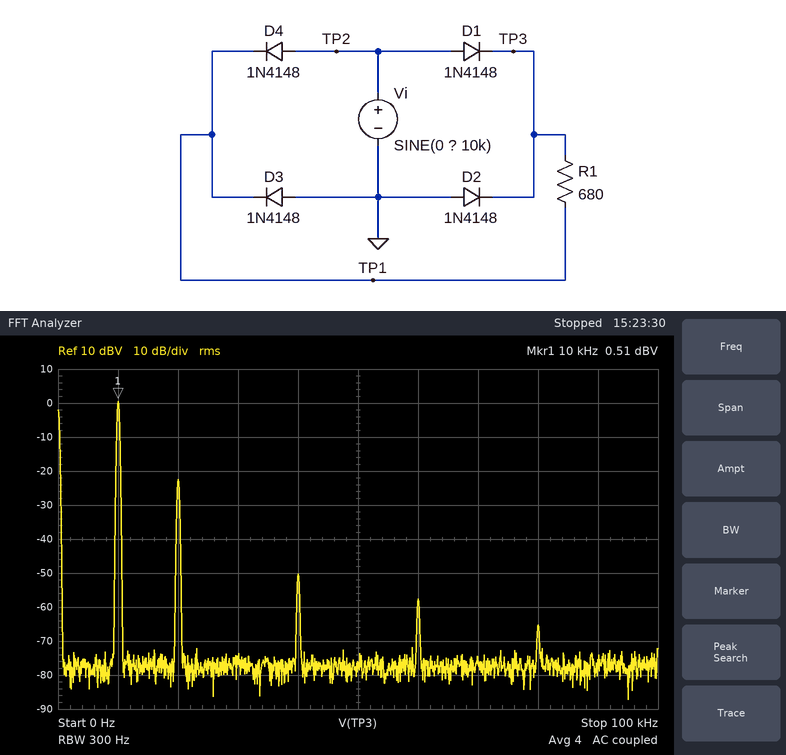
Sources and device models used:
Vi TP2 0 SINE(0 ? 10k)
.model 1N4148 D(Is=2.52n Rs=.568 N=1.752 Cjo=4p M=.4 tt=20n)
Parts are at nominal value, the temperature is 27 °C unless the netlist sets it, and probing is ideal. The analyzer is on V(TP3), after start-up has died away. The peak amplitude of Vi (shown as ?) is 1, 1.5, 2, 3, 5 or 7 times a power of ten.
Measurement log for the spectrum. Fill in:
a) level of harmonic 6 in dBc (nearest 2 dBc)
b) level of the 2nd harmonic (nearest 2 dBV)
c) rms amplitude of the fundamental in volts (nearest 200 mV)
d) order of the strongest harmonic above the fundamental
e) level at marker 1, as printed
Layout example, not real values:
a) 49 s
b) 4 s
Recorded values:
a) -58 dBc
b) -22 dBV
c) 1.0 V
d) 2
e) 0.51 dBV
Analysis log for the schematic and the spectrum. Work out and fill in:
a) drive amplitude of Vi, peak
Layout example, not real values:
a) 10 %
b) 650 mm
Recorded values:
a) 3 V
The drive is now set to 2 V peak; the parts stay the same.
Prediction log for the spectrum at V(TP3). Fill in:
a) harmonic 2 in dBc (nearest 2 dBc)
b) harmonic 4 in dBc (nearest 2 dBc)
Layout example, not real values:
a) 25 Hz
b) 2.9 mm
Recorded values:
a) -24 dBc
b) -48 dBc
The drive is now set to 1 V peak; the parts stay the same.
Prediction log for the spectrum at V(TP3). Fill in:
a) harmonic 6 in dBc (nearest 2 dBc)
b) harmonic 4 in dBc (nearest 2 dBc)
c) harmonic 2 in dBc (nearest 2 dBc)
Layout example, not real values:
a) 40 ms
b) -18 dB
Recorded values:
a) -60 dBc
b) -46 dBc
c) -28 dBc
